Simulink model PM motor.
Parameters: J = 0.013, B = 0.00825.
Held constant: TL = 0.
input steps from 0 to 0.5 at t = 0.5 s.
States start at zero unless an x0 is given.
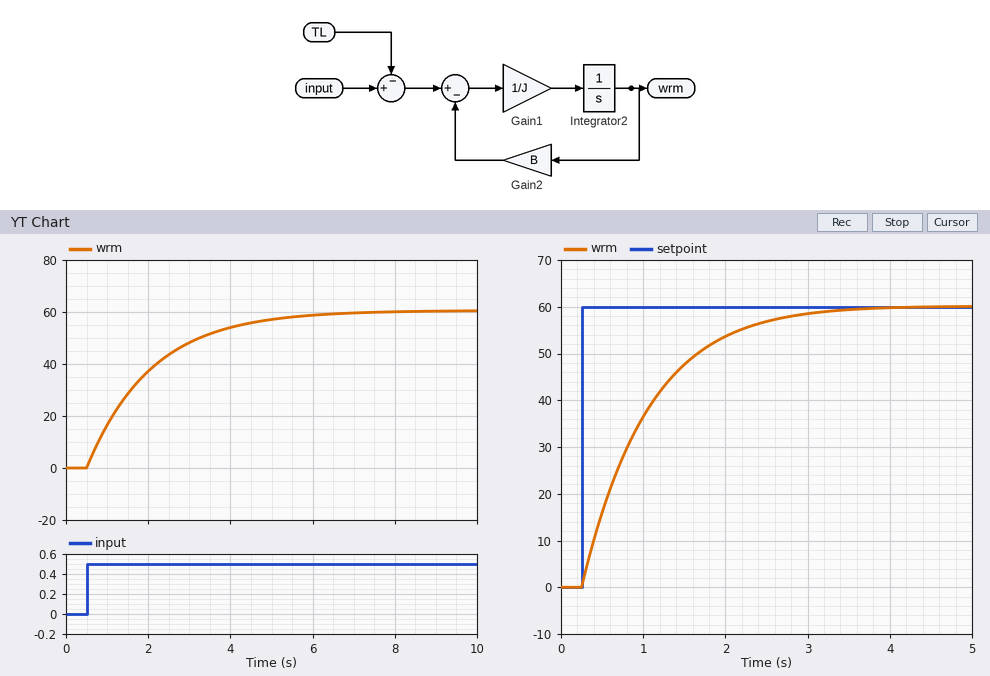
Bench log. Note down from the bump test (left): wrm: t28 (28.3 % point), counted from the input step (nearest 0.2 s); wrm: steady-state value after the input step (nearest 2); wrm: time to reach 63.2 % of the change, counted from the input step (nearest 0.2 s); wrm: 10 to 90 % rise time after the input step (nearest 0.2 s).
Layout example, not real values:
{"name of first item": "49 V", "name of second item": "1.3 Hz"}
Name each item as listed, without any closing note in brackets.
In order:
{"wrm: t28 (28.3 % point), counted from the input step": "0.6 s", "wrm: steady-state value after the input step": "60", "wrm: time to reach 63.2 % of the change, counted from the input step": "1.6 s", "wrm: 10 to 90 % rise time after the input step": "3.4 s"}
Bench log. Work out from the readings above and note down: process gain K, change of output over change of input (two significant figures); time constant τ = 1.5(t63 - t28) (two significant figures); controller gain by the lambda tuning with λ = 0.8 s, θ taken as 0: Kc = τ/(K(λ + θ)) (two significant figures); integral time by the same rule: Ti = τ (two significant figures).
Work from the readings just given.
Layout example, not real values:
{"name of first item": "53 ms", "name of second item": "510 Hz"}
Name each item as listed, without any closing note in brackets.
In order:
{"process gain K, change of output over change of input": "120", "time constant τ = 1.5(t63 - t28)": "1.5 s", "controller gain by the lambda tuning with λ = 0.8 s, θ taken as 0: Kc = τ/(K(λ + θ))": "0.016", "integral time by the same rule: Ti = τ": "1.5 s"}
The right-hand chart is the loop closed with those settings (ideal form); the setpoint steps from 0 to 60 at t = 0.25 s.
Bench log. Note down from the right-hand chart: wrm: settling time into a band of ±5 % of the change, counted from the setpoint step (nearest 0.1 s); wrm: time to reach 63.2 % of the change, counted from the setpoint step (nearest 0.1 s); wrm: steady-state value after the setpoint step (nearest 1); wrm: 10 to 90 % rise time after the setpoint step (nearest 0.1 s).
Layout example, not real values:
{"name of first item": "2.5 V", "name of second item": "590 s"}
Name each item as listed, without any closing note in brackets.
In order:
{"wrm: settling time into a band of ±5 % of the change, counted from the setpoint step": "2.3 s", "wrm: time to reach 63.2 % of the change, counted from the setpoint step": "0.8 s", "wrm: steady-state value after the setpoint step": "60", "wrm: 10 to 90 % rise time after the setpoint step": "1.7 s"}
